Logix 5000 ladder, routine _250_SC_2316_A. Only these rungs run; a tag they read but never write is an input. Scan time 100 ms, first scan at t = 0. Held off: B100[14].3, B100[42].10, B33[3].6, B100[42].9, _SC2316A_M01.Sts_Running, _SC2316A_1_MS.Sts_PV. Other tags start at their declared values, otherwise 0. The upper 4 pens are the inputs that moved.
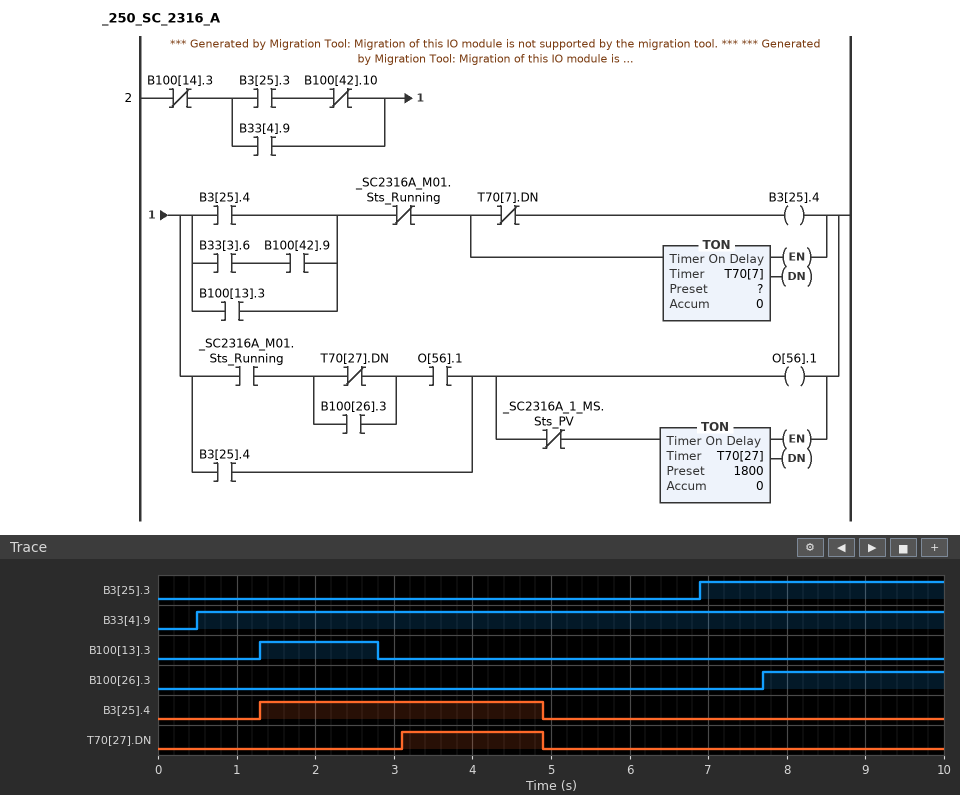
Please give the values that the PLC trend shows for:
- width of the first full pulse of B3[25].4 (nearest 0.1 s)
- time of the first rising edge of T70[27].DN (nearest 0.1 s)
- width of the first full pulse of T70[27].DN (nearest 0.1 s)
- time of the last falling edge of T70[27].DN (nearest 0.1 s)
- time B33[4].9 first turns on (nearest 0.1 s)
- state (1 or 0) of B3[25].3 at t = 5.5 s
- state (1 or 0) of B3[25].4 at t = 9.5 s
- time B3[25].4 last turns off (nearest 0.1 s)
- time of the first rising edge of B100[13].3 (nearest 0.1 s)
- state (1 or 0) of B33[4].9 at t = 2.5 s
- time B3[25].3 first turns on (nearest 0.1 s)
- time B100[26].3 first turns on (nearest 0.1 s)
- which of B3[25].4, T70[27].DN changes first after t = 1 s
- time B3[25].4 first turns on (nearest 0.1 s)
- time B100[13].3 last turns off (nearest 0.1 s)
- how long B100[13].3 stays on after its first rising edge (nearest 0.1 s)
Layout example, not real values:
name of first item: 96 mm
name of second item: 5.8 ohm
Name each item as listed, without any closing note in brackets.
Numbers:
width of the first full pulse of B3[25].4: 3.6 s
time of the first rising edge of T70[27].DN: 3.1 s
width of the first full pulse of T70[27].DN: 1.8 s
time of the last falling edge of T70[27].DN: 4.9 s
time B33[4].9 first turns on: 0.5 s
state (1 or 0) of B3[25].3 at t = 5.5 s: 0
state (1 or 0) of B3[25].4 at t = 9.5 s: 0
time B3[25].4 last turns off: 4.9 s
time of the first rising edge of B100[13].3: 1.3 s
state (1 or 0) of B33[4].9 at t = 2.5 s: 1
time B3[25].3 first turns on: 6.9 s
time B100[26].3 first turns on: 7.7 s
which of B3[25].4, T70[27].DN changes first after t = 1 s: B3[25].4
time B3[25].4 first turns on: 1.3 s
time B100[13].3 last turns off: 2.8 s
how long B100[13].3 stays on after its first rising edge: 1.5 s
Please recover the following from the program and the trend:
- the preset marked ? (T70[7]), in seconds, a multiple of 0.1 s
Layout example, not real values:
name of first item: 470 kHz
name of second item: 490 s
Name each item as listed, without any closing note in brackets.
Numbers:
the preset marked ? (T70[7]), in seconds, a multiple of 0.1 s: 3.5 s
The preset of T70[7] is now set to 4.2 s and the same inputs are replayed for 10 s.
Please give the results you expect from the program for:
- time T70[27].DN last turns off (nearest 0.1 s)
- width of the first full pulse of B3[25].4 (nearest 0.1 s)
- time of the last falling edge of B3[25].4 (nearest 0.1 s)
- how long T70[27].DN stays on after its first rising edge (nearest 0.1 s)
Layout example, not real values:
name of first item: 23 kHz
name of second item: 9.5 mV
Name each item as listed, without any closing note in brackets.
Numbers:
time T70[27].DN last turns off: 5.6 s
width of the first full pulse of B3[25].4: 4.3 s
time of the last falling edge of B3[25].4: 5.6 s
how long T70[27].DN stays on after its first rising edge: 2.5 s
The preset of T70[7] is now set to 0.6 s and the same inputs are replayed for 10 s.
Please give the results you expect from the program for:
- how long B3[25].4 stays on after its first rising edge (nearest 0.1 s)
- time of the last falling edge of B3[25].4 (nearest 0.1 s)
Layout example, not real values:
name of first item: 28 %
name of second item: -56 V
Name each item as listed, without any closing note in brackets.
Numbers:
how long B3[25].4 stays on after its first rising edge: 0.7 s
time of the last falling edge of B3[25].4: 2.0 s
